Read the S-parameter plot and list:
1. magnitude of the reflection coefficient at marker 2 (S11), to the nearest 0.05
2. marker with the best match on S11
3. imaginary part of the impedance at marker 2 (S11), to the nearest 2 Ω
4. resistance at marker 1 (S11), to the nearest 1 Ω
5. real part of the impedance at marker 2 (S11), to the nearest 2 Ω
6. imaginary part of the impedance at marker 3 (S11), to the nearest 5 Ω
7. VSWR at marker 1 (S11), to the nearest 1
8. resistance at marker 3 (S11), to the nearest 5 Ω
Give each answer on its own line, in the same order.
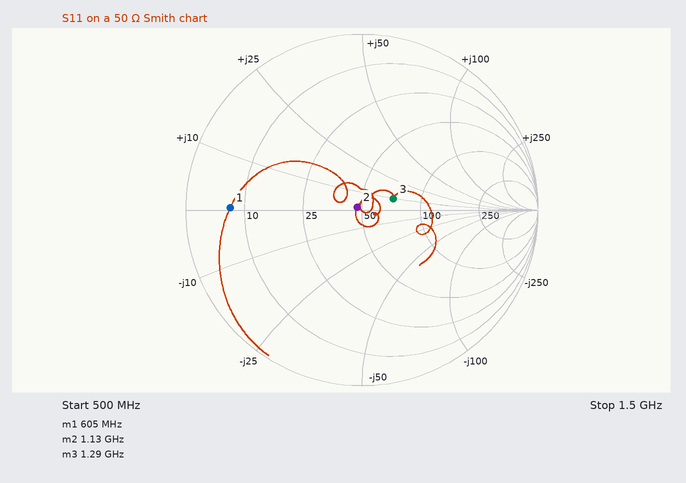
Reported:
0.05
marker 2
+2 Ω
7 Ω
48 Ω
+10 Ω
7
70 Ω
